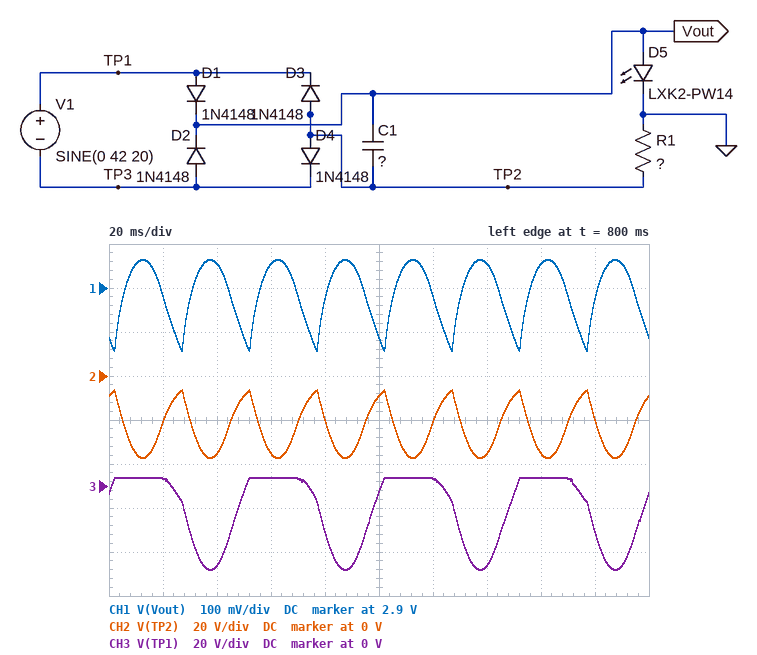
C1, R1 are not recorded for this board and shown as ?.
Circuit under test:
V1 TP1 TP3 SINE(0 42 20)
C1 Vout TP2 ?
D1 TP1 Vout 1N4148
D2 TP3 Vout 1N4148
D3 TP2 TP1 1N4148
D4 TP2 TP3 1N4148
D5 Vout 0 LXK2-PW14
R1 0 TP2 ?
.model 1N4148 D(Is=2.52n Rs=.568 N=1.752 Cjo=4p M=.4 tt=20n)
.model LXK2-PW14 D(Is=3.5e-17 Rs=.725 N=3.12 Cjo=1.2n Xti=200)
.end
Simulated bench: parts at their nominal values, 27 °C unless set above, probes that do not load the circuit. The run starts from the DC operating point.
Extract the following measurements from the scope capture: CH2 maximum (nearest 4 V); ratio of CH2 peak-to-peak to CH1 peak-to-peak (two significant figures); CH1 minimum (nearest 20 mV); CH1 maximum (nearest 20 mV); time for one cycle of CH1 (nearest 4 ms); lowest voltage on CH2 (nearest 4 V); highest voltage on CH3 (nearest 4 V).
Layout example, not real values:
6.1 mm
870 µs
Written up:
-8 V
150
2.76 V
2.96 V
24 ms
-36 V
4 V
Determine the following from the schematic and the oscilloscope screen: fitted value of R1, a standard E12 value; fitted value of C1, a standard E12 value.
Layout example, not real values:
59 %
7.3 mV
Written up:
330 Ω
18 µF
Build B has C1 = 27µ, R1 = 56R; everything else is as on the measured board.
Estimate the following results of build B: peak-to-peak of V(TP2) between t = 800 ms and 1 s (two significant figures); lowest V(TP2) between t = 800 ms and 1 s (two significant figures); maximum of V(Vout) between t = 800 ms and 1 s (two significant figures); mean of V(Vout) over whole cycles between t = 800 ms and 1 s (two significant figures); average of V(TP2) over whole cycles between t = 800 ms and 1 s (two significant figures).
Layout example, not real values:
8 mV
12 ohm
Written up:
35 V
-36 V
3.5 V
3.2 V
-22 V
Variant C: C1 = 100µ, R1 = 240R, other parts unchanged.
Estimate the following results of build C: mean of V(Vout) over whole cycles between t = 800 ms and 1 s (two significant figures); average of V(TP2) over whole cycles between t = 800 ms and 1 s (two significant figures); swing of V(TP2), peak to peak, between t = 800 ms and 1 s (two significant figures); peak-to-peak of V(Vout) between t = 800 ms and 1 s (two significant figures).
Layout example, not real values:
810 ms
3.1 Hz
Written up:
3.0 V
-29 V
18 V
110 mV
